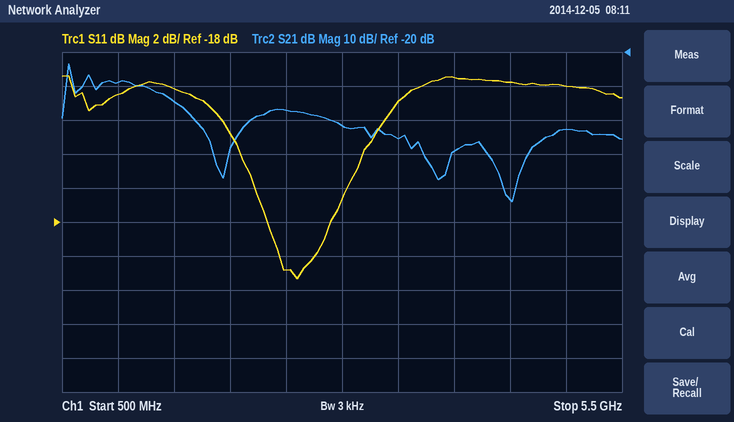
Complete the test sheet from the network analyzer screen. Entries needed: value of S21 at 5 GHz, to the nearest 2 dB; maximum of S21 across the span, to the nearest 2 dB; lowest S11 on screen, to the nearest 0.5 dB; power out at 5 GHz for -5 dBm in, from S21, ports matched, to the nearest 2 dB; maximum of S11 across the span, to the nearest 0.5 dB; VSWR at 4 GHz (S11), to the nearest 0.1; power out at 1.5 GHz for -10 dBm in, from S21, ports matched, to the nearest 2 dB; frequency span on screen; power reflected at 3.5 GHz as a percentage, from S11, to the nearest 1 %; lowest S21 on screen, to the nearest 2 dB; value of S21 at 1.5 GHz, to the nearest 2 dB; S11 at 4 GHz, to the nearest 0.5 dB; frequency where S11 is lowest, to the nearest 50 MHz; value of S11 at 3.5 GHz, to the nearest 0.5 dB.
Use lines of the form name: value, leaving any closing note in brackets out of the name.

value of S21 at 5 GHz, to the nearest 2 dB: -42 dB
maximum of S21 across the span, to the nearest 2 dB: -24 dB
lowest S11 on screen, to the nearest 0.5 dB: -21.5 dB
power out at 5 GHz for -5 dBm in, from S21, ports matched, to the nearest 2 dB: -48 dBm
maximum of S11 across the span, to the nearest 0.5 dB: -9.5 dB
VSWR at 4 GHz (S11), to the nearest 0.1: 2.0
power out at 1.5 GHz for -10 dBm in, from S21, ports matched, to the nearest 2 dB: -44 dBm
frequency span on screen: 5 GHz
power reflected at 3.5 GHz as a percentage, from S11, to the nearest 1 %: 8 %
lowest S21 on screen, to the nearest 2 dB: -64 dB
value of S21 at 1.5 GHz, to the nearest 2 dB: -34 dB
S11 at 4 GHz, to the nearest 0.5 dB: -9.5 dB
frequency where S11 is lowest, to the nearest 50 MHz: 2.60 GHz
value of S11 at 3.5 GHz, to the nearest 0.5 dB: -11.0 dB
